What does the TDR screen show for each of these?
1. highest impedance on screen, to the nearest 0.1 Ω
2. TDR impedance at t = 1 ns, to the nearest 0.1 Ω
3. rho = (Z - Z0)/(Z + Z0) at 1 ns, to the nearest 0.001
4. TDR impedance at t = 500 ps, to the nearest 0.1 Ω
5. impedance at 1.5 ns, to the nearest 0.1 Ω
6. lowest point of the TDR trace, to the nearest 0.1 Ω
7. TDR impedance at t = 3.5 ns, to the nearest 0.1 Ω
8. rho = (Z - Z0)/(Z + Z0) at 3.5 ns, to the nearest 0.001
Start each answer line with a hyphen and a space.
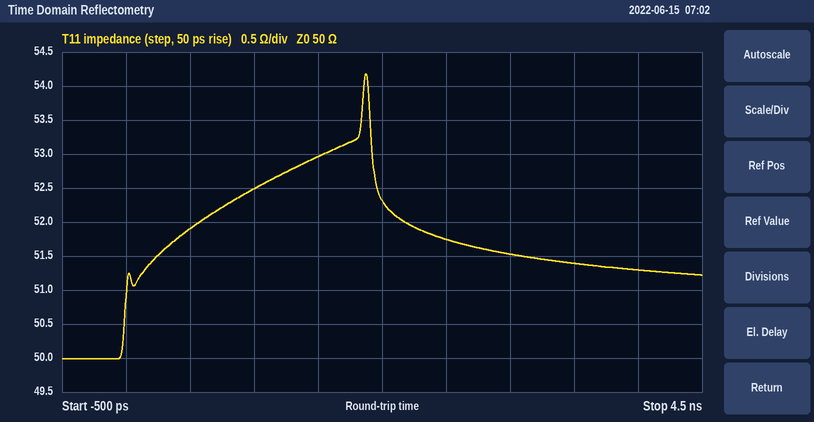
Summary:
- 54.2 Ω
- 52.5 Ω
- +0.024
- 51.9 Ω
- 53.0 Ω
- 50.0 Ω
- 51.4 Ω
- +0.014
